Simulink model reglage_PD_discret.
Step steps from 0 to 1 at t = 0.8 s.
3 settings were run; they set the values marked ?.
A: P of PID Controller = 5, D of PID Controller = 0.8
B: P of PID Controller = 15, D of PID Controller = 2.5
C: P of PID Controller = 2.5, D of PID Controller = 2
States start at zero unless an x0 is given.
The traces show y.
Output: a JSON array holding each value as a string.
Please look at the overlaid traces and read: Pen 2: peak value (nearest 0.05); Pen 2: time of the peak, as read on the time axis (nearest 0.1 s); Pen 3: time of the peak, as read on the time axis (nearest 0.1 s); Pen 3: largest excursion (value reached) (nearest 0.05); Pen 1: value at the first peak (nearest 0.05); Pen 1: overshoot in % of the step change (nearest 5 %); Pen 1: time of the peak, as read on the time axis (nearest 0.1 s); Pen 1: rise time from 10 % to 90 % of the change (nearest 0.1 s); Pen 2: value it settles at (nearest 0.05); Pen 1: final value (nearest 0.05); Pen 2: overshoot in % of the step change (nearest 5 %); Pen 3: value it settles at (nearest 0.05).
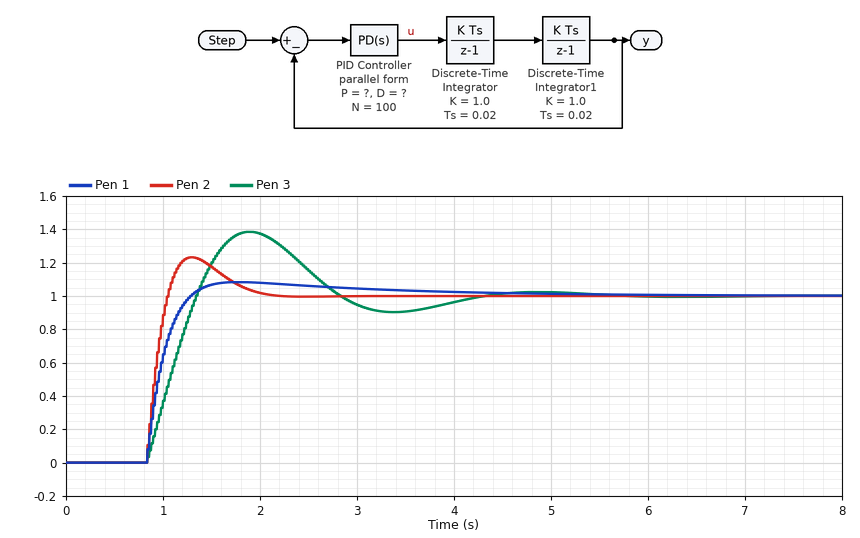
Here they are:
["1.25", "1.3 s", "1.9 s", "1.40", "1.10", "10 %", "1.8 s", "0.3 s", "1.00", "1.00", "25 %", "1.00"]
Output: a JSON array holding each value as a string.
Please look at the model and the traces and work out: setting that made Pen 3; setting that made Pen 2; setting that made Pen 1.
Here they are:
["A", "B", "C"]
